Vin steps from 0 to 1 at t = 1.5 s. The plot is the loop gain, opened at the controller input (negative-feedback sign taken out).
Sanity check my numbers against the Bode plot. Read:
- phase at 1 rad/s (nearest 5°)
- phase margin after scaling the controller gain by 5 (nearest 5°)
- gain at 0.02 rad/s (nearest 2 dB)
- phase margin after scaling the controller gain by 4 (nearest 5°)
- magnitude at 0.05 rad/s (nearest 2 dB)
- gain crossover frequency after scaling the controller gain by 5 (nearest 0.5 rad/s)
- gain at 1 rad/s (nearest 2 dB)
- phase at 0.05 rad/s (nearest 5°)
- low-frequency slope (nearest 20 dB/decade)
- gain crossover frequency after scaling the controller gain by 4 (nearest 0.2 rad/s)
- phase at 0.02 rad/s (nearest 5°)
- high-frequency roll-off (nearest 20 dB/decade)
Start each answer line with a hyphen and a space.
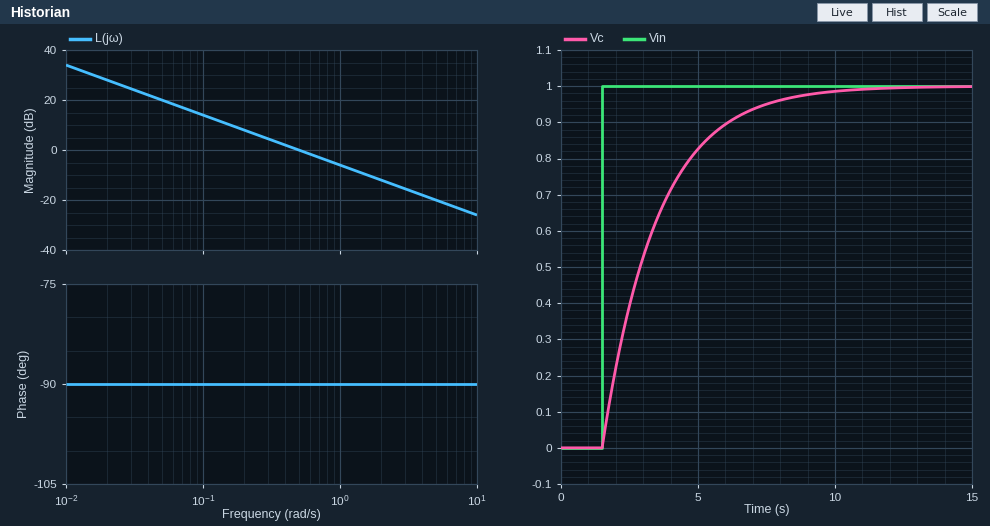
- -90°
- 90°
- 28 dB
- 90°
- 20 dB
- 2.5 rad/s
- -6 dB
- -90°
- -20 dB/decade
- 2.0 rad/s
- -90°
- -20 dB/decade
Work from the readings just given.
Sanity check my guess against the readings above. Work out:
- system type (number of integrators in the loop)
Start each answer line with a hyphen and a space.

- 1
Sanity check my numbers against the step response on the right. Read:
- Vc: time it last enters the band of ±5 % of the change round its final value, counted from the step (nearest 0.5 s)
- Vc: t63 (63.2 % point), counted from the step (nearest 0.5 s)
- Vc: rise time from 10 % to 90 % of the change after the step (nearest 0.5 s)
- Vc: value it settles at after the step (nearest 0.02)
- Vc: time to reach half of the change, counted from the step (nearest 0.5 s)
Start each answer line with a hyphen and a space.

- 6.0 s
- 2.0 s
- 4.5 s
- 1.00
- 1.5 s
